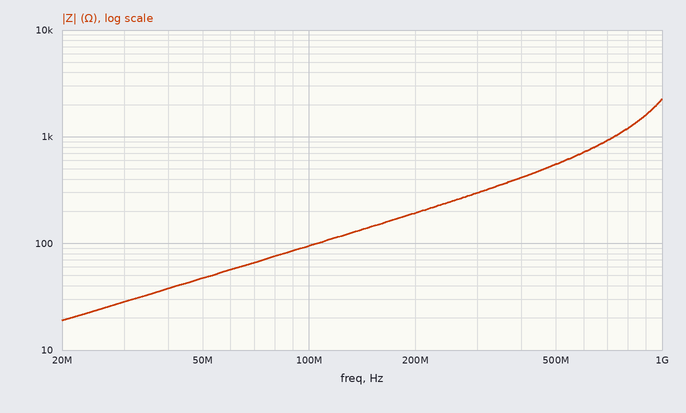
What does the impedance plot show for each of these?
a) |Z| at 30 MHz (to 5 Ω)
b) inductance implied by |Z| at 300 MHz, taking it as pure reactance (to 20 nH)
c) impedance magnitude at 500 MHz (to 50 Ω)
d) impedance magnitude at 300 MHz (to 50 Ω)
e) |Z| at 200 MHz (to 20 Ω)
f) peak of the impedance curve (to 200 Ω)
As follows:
30 Ω
160 nH
550 Ω
300 Ω
200 Ω
2.2 kΩ
